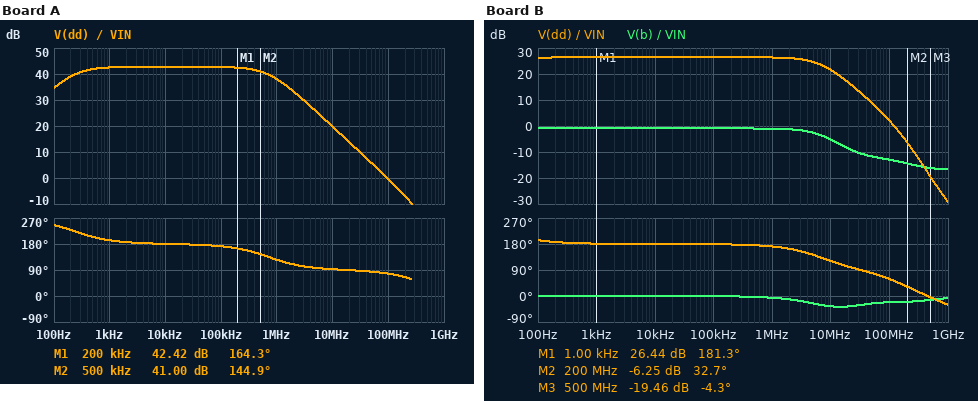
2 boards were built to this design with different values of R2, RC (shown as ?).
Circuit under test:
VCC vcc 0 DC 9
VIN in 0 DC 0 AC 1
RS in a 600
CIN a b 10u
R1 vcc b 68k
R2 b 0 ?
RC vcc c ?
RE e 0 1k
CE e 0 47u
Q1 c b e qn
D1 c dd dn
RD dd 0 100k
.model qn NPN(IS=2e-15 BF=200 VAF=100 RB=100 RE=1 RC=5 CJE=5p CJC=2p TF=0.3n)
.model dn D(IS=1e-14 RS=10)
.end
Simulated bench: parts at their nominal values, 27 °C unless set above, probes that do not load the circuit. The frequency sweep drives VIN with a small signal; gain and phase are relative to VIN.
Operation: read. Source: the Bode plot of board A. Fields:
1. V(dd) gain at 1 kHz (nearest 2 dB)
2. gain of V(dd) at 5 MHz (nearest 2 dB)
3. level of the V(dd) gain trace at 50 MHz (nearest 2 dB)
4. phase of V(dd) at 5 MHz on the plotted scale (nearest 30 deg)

42 dB
26 dB
6 dB
90 deg
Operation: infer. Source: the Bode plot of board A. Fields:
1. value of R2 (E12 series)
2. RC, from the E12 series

47 kΩ
2.2 kΩ
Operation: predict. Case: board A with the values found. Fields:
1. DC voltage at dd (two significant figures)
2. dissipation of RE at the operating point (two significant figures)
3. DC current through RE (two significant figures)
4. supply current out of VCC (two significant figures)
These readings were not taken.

2.7 V
6.7 mW
2.6 mA
2.7 mA
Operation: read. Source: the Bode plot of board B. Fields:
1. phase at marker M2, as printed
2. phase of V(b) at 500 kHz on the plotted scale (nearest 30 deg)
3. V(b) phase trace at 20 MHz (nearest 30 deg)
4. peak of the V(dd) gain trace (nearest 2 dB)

32.7 deg
0 deg
-30 deg
26 dB
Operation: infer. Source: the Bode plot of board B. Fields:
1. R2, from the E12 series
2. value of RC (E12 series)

6.8 kΩ
3.9 kΩ
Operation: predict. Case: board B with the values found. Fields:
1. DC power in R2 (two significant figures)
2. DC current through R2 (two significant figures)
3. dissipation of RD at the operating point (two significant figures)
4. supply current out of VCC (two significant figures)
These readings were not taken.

97 µW
120 µA
560 µW
360 µA
